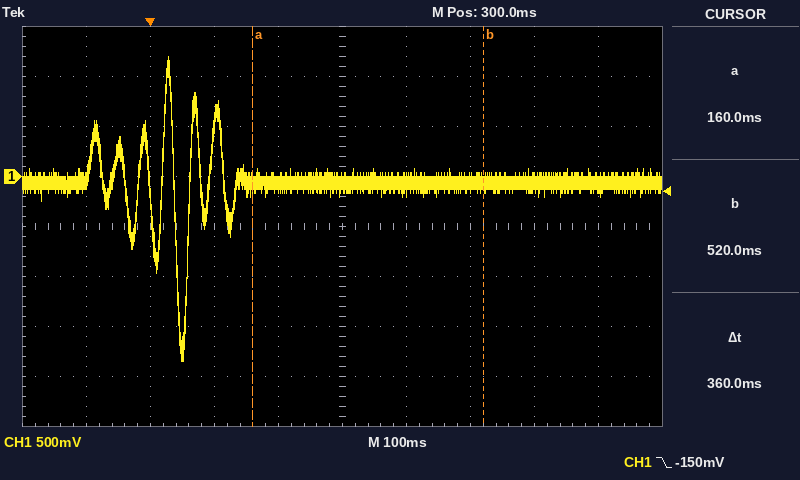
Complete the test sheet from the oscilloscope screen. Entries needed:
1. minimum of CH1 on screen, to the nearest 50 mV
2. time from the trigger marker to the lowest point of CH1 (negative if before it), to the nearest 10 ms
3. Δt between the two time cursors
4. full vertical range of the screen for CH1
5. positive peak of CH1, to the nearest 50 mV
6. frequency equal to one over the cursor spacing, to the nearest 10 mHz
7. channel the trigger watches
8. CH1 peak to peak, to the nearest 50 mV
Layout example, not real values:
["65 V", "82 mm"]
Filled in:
["-1.85 V", "+50 ms", "360 ms", "4 V", "1.20 V", "2.78 Hz", "CH1", "3.05 V"]
